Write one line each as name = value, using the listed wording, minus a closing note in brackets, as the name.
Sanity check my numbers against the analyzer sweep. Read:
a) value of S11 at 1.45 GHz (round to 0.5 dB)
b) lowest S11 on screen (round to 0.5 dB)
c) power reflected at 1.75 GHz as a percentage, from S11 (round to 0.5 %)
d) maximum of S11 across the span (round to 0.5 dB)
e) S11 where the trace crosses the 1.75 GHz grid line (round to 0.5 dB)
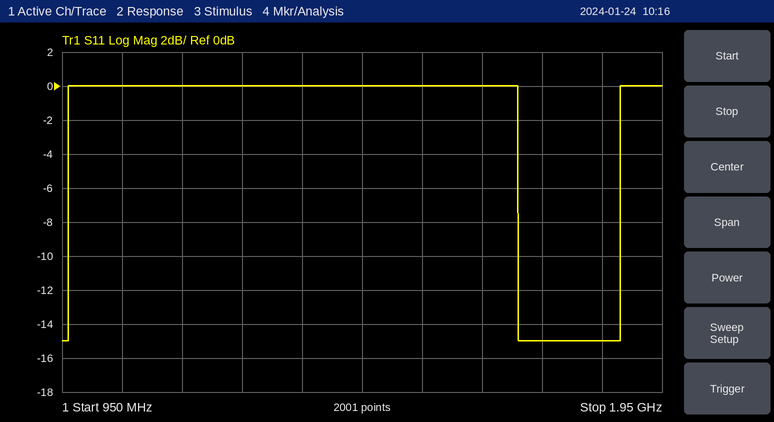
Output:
value of S11 at 1.45 GHz = 0.0 dB
lowest S11 on screen = -15.0 dB
power reflected at 1.75 GHz as a percentage, from S11 = 3.0 %
maximum of S11 across the span = 0.0 dB
S11 where the trace crosses the 1.75 GHz grid line = -15.0 dB
